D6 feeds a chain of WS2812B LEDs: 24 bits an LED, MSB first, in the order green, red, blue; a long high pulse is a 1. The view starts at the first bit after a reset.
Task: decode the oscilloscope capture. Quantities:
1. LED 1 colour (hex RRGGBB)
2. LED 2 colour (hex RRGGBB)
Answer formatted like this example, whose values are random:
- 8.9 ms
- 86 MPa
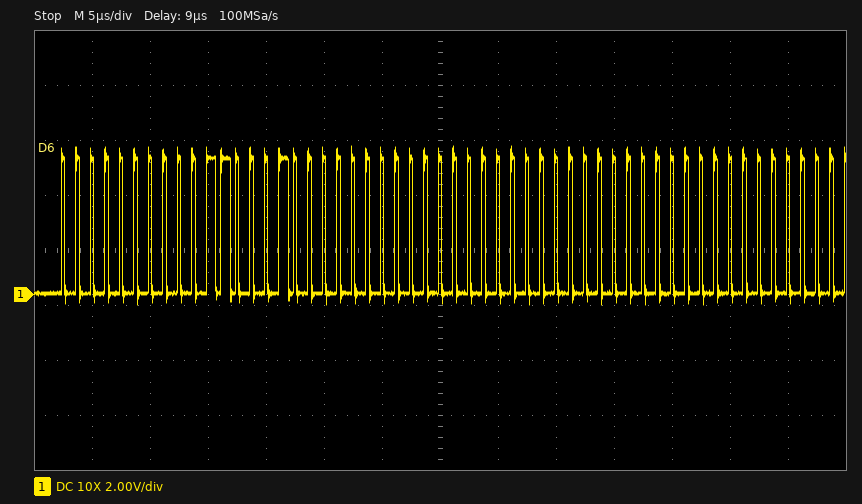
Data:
- #310000
- #000000
